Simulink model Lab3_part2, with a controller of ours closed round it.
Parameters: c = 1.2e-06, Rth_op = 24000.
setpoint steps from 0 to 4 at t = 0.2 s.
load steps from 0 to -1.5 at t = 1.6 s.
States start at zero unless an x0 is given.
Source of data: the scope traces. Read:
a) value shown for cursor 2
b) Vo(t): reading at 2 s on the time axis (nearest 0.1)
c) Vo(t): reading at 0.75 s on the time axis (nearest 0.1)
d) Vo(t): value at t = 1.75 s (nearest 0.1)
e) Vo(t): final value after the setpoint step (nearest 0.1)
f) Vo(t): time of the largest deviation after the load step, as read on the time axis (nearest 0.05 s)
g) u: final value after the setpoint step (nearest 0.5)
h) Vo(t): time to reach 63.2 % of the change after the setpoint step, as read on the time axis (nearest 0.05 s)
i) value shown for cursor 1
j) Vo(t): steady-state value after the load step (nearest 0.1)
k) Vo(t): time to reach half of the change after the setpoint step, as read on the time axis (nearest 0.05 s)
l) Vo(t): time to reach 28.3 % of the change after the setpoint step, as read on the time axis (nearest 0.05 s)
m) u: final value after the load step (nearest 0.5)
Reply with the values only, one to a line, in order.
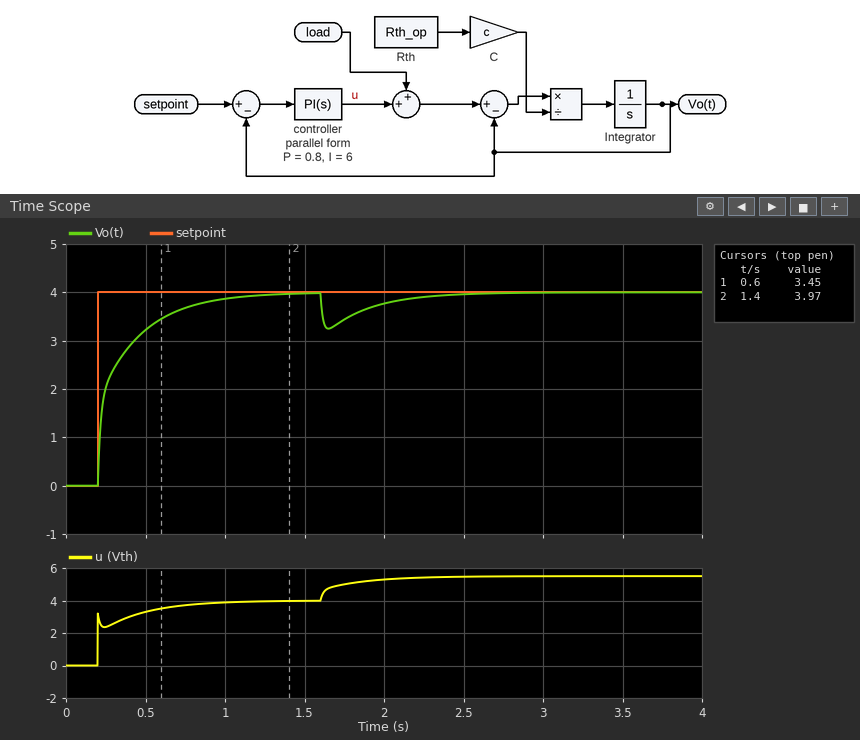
3.97
3.8
3.7
3.4
4.0
1.65 s
4.0
0.30 s
3.45
4.0
0.25 s
0.20 s
5.5
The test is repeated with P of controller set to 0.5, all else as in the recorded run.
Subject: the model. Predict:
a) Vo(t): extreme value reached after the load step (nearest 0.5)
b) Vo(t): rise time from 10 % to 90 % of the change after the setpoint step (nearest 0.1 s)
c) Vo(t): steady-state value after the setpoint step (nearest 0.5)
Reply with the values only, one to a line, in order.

3.0
0.4 s
4.0
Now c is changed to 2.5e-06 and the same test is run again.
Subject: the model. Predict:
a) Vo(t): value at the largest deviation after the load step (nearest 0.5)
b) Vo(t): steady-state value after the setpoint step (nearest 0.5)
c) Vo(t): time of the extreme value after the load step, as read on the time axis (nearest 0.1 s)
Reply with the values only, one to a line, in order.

3.5
4.0
1.7 s
